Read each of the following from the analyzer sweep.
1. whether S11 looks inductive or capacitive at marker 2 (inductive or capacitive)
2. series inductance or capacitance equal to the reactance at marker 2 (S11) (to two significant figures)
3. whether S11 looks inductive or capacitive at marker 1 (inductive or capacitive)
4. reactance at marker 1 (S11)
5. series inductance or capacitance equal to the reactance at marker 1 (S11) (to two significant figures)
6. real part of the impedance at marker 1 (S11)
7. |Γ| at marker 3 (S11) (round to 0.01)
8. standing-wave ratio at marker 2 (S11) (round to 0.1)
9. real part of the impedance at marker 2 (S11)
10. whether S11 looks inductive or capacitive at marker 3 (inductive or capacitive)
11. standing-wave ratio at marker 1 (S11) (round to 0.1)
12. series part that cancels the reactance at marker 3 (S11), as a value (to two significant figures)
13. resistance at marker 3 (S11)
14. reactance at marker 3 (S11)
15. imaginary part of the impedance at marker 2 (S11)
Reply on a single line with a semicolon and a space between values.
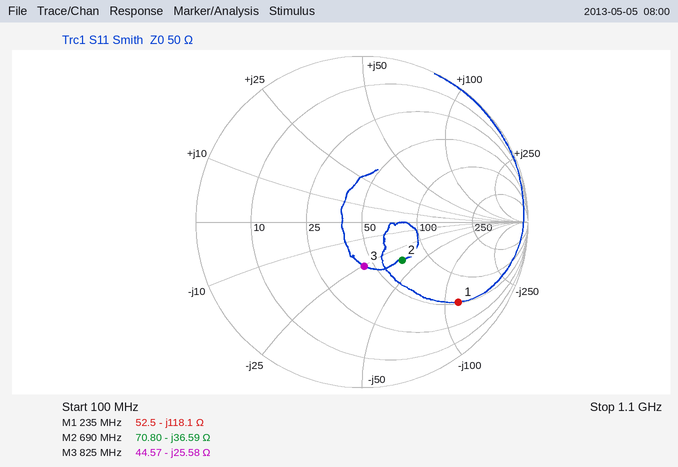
capacitive; 6.3 pF; capacitive; -118.1 Ω; 5.7 pF; 52.5 Ω; 0.27; 2.0; 70.80 Ω; capacitive; 7.2; 4.9 nH; 44.57 Ω; -25.58 Ω; -36.59 Ω
